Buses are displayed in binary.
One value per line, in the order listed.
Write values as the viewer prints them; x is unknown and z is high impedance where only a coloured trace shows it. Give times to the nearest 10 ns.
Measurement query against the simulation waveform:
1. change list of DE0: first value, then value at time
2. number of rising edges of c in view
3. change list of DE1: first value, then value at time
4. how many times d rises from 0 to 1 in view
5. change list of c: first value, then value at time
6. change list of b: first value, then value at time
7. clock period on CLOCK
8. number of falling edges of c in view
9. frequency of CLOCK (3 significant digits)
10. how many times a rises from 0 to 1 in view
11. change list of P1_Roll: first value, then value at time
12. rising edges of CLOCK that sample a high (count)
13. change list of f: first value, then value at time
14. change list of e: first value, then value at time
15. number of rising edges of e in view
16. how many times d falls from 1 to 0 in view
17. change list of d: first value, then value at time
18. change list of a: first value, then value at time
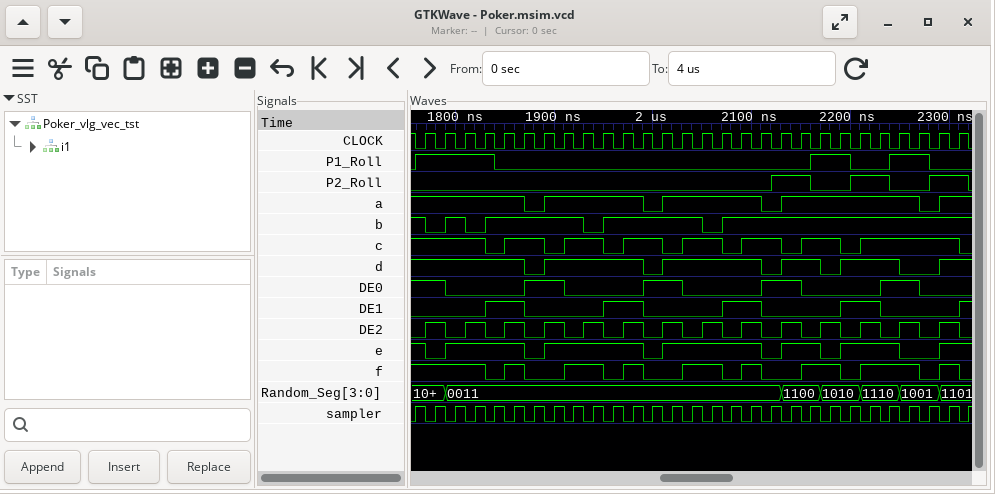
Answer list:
1, 0 at 1790 ns, 1 at 1870 ns, 0 at 1910 ns, 1 at 1990 ns, 0 at 2030 ns, 1 at 2110 ns, 0 at 2150 ns, 1 at 2230 ns, 0 at 2270 ns
7
0, 1 at 1830 ns, 0 at 1870 ns, 1 at 1950 ns, 0 at 1990 ns, 1 at 2070 ns, 0 at 2110 ns, 1 at 2190 ns, 0 at 2230 ns, 1 at 2310 ns
5
1, 0 at 1830 ns, 1 at 1850 ns, 0 at 1890 ns, 1 at 1910 ns, 0 at 1950 ns, 1 at 1970 ns, 0 at 2010 ns, 1 at 2030 ns, 0 at 2070 ns, 1 at 2090 ns, 0 at 2130 ns, 1 at 2150 ns, 0 at 2190 ns, 1 at 2210 ns, 0 at 2310 ns
1, 0 at 1770 ns, 1 at 1790 ns, 0 at 1810 ns, 1 at 1830 ns, 0 at 1930 ns, 1 at 1950 ns, 0 at 2050 ns, 1 at 2070 ns
20 ns
8
50.0 MHz
4
0, 1 at 1760 ns, 0 at 1840 ns, 1 at 2160 ns, 0 at 2200 ns, 1 at 2240 ns, 0 at 2280 ns
24
1, 0 at 1830 ns, 1 at 1850 ns, 0 at 1870 ns, 1 at 1910 ns, 0 at 1950 ns, 1 at 1970 ns, 0 at 1990 ns, 1 at 2030 ns, 0 at 2070 ns, 1 at 2090 ns, 0 at 2110 ns, 1 at 2150 ns, 0 at 2190 ns, 1 at 2210 ns, 0 at 2270 ns, 1 at 2290 ns, 0 at 2310 ns
1, 0 at 1770 ns, 1 at 1790 ns, 0 at 1870 ns, 1 at 1890 ns, 0 at 1990 ns, 1 at 2010 ns, 0 at 2110 ns, 1 at 2130 ns, 0 at 2170 ns, 1 at 2190 ns, 0 at 2250 ns, 1 at 2290 ns
6
5
1, 0 at 1870 ns, 1 at 1890 ns, 0 at 1990 ns, 1 at 2010 ns, 0 at 2110 ns, 1 at 2130 ns, 0 at 2170 ns, 1 at 2190 ns, 0 at 2250 ns, 1 at 2290 ns
1, 0 at 1870 ns, 1 at 1890 ns, 0 at 1990 ns, 1 at 2010 ns, 0 at 2110 ns, 1 at 2130 ns, 0 at 2270 ns, 1 at 2290 ns
